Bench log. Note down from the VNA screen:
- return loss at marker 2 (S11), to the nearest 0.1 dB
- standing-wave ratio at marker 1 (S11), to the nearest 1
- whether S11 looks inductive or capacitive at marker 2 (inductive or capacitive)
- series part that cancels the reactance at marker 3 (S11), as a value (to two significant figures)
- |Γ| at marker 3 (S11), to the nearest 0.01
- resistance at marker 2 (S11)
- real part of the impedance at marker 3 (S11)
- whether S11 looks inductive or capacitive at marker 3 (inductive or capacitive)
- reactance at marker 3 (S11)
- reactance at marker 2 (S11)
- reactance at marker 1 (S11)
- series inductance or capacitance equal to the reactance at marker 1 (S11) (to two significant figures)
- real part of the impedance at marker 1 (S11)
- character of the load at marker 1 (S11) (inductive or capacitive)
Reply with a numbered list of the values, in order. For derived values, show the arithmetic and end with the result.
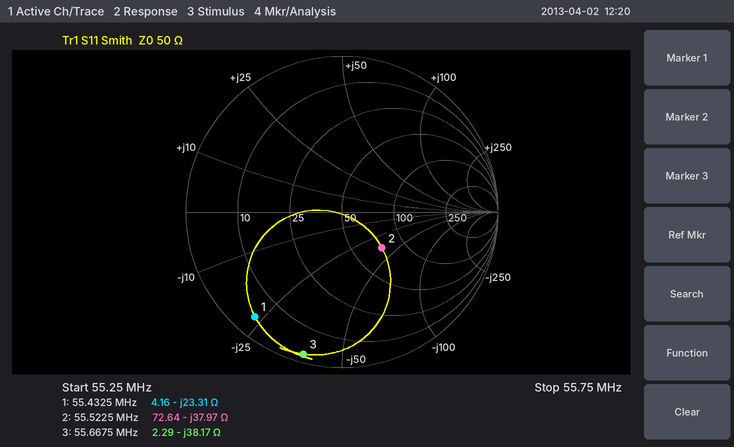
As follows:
1. 9.3 dB
2. 15
3. capacitive
4. L = 38.17 Ω/(2π × 55.6675 MHz) ≈ 109 nH, so 110 nH to two significant figures
5. 0.94
6. 72.64 Ω
7. 2.29 Ω
8. capacitive
9. -38.17 Ω
10. -37.97 Ω
11. -23.31 Ω
12. C = 1/(2π × 55.4325 MHz × 23.31 Ω) ≈ 123 pF, so 120 pF to two significant figures
13. 4.16 Ω
14. capacitive
